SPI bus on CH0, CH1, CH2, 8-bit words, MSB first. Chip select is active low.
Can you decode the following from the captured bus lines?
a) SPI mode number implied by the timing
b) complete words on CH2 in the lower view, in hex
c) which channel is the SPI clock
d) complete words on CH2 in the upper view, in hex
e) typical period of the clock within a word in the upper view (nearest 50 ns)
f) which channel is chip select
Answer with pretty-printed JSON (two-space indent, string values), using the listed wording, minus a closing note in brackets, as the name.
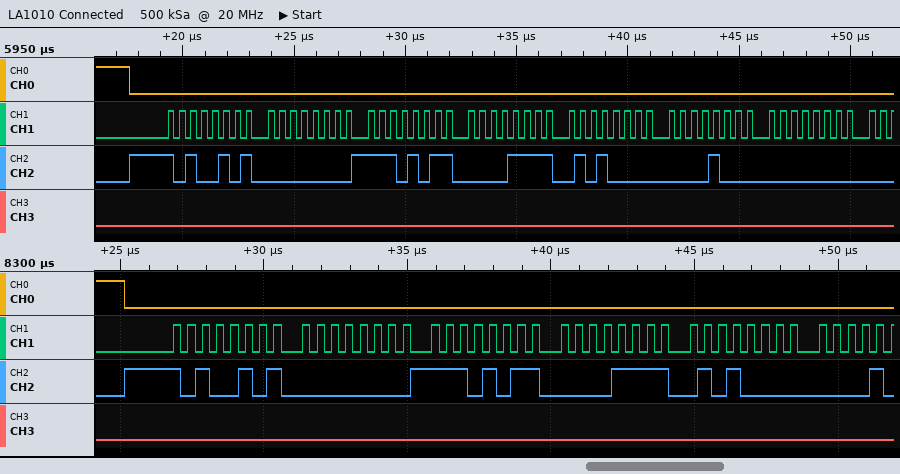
{
  "SPI mode number implied by the timing": "0",
  "complete words on CH2 in the lower view, in hex": "A5, 00, EB, 0F, 50",
  "which channel is the SPI clock": "CH1",
  "complete words on CH2 in the upper view, in hex": "A5, 00, EB, 0F, 50, 08, 00",
  "typical period of the clock within a word in the upper view": "500 ns",
  "which channel is chip select": "CH0"
}
